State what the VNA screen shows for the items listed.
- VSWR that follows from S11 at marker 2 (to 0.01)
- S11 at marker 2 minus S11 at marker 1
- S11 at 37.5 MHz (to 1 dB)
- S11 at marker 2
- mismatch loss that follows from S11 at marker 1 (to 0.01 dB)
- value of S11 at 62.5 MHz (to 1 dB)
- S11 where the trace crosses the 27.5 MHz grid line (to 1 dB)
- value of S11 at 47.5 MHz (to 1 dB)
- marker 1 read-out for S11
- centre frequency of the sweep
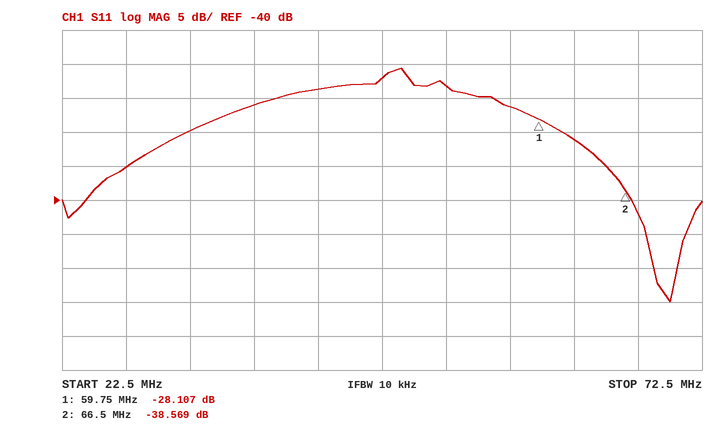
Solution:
1.02
-10.462 dB
-26 dB
-38.569 dB
0.01 dB
-31 dB
-35 dB
-22 dB
-28.107 dB
47.5 MHz
